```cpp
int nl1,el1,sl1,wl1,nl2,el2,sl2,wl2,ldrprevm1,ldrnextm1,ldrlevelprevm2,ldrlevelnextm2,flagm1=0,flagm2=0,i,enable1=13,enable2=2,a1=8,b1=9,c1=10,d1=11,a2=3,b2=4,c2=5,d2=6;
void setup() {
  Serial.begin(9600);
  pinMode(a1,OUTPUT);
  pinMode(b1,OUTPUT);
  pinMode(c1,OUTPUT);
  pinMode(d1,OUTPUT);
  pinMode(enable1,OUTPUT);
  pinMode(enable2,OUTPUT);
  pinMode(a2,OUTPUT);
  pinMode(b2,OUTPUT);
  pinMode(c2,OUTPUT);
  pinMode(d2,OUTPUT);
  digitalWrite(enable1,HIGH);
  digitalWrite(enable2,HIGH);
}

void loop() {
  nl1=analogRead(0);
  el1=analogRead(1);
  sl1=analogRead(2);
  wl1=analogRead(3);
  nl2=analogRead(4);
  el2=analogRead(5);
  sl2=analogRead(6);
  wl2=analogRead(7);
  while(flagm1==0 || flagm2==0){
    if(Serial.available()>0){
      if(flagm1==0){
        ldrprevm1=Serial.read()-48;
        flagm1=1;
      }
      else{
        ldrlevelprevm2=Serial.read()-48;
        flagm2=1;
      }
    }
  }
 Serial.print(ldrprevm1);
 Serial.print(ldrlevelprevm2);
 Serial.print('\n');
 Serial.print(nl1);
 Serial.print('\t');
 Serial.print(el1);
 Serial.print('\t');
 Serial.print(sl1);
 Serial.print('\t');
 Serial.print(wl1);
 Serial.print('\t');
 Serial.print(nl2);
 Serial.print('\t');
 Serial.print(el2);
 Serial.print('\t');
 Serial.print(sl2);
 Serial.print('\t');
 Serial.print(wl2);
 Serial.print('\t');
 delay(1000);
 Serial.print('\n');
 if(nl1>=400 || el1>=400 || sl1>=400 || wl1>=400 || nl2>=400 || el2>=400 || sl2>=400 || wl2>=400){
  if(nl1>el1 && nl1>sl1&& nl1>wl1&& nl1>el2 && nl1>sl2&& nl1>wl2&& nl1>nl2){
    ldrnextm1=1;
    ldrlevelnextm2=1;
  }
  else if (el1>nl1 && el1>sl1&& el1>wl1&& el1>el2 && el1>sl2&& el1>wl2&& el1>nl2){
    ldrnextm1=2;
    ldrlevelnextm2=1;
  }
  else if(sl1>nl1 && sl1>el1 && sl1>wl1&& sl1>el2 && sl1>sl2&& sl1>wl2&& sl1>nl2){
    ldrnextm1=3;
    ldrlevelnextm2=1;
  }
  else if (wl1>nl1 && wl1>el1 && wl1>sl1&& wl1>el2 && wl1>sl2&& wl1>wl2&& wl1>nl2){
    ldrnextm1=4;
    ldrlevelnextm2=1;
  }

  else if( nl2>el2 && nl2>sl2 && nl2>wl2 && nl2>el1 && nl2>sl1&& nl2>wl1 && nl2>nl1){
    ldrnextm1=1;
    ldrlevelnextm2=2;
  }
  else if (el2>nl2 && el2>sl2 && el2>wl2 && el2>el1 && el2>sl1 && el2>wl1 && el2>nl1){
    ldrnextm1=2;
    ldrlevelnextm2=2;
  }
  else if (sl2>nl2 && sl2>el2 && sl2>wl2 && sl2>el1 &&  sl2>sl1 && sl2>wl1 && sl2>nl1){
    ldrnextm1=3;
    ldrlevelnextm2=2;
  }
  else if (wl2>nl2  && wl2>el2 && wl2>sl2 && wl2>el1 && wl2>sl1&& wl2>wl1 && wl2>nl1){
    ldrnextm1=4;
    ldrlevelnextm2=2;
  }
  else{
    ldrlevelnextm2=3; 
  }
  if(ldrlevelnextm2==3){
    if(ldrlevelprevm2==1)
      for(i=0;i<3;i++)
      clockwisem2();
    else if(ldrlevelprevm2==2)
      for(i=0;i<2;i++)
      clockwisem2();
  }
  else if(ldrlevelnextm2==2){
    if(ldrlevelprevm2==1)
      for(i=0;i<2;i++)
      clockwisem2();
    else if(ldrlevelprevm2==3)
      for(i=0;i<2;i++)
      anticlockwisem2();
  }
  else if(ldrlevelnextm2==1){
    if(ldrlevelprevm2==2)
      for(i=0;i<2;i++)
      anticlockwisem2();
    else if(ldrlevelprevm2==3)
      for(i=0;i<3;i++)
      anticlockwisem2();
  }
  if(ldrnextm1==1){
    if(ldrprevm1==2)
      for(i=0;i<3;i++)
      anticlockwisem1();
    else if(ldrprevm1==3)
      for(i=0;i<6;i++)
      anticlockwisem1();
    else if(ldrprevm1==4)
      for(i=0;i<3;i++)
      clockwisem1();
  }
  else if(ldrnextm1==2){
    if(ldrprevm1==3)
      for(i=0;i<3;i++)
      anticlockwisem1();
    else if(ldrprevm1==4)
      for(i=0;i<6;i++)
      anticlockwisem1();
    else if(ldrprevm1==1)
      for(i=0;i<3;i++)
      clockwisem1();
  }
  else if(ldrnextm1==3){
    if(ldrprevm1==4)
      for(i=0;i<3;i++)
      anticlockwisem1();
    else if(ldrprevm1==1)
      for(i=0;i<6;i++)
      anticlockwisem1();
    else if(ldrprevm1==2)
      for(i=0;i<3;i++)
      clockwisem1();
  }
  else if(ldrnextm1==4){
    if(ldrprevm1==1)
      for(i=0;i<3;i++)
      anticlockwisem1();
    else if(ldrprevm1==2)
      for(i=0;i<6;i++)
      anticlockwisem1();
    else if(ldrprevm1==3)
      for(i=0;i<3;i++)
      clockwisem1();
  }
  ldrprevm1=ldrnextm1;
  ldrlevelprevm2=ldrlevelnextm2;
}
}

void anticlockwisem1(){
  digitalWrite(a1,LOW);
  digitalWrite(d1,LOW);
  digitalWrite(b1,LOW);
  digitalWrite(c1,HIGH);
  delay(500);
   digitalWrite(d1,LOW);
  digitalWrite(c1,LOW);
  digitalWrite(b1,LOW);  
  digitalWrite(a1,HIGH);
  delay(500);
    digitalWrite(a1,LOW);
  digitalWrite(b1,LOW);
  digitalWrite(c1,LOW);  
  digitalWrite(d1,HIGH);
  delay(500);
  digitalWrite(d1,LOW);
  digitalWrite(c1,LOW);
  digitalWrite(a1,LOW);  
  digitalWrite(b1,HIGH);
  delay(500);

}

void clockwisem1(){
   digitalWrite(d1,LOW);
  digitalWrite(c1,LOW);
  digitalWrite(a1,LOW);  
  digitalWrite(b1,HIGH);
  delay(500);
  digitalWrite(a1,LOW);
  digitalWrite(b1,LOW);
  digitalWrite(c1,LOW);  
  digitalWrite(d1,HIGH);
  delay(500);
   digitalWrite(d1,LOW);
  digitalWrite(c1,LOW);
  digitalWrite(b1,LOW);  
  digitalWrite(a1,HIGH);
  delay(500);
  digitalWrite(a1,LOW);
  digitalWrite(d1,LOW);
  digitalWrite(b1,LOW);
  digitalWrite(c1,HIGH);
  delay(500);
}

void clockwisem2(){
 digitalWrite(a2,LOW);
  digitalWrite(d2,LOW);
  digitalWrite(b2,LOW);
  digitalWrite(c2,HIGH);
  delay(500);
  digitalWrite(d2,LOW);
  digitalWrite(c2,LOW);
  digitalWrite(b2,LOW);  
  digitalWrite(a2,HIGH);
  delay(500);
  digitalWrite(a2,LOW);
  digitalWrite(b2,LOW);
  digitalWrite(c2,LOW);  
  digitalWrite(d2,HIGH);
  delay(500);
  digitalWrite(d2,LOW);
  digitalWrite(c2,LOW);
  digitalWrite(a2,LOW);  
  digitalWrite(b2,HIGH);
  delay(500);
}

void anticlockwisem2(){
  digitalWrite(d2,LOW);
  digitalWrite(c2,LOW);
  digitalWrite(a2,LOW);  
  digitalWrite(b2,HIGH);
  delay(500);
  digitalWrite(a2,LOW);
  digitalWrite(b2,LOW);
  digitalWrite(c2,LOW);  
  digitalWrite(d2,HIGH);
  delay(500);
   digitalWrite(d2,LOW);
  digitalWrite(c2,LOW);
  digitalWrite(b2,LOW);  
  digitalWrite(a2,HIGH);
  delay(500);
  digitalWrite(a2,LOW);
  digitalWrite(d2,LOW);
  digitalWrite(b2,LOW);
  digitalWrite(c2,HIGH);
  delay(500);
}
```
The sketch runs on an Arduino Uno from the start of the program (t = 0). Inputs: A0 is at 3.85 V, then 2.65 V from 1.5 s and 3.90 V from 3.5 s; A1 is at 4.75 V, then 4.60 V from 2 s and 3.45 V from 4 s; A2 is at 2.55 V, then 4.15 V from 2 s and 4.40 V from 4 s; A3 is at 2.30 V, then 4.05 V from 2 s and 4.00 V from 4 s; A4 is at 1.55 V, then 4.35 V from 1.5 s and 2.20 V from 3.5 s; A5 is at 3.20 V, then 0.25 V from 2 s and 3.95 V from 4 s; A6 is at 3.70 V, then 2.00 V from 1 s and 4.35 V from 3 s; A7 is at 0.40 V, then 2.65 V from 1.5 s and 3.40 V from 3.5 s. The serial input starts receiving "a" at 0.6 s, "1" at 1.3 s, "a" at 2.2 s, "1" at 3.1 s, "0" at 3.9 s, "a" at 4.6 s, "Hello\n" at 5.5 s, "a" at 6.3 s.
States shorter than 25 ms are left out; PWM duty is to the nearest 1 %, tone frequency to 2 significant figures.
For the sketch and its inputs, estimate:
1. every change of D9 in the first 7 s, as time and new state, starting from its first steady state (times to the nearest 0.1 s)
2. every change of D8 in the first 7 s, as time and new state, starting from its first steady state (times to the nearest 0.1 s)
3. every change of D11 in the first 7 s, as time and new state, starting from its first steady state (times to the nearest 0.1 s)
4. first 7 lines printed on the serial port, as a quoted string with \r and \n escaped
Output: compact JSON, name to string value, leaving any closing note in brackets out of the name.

{"every change of D9 in the first 7 s, as time and new state, starting from its first steady state": "0 s low; 5.3 s high; 5.8 s low", "every change of D8 in the first 7 s, as time and new state, starting from its first steady state": "0 s low; 6.3 s high; 6.8 s low", "every change of D11 in the first 7 s, as time and new state, starting from its first steady state": "0 s low; 5.8 s high; 6.3 s low", "first 7 lines printed on the serial port, as a quoted string with \\r and \\n escaped": "\"491\\n788\\t972\\t522\\t471\\t317\\t655\\t757\\t81\\t\\n21\\n542\\t942\\t849\\t829\\t890\\t51\\t409\\t542\\t\\n21\\n542\\t942\\t849\\t829\\t890\\t51\\t890\\t542\\t\\n21\\n\""}
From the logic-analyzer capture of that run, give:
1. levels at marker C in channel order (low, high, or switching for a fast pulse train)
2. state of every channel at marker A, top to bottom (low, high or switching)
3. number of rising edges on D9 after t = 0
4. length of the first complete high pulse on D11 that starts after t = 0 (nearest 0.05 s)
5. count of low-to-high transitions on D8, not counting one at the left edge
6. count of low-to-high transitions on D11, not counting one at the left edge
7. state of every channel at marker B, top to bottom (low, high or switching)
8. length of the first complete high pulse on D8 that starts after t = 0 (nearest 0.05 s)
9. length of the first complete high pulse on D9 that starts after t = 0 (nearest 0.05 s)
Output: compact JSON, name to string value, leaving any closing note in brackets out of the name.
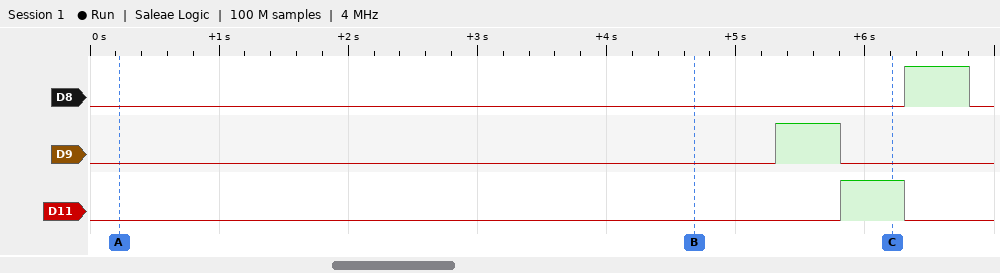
{"levels at marker C in channel order": "D8 low, D9 low, D11 high", "state of every channel at marker A, top to bottom": "D8 low, D9 low, D11 low", "number of rising edges on D9 after t = 0": "1", "length of the first complete high pulse on D11 that starts after t = 0": "0.50 s", "count of low-to-high transitions on D8, not counting one at the left edge": "1", "count of low-to-high transitions on D11, not counting one at the left edge": "1", "state of every channel at marker B, top to bottom": "D8 low, D9 low, D11 low", "length of the first complete high pulse on D8 that starts after t = 0": "0.50 s", "length of the first complete high pulse on D9 that starts after t = 0": "0.50 s"}
